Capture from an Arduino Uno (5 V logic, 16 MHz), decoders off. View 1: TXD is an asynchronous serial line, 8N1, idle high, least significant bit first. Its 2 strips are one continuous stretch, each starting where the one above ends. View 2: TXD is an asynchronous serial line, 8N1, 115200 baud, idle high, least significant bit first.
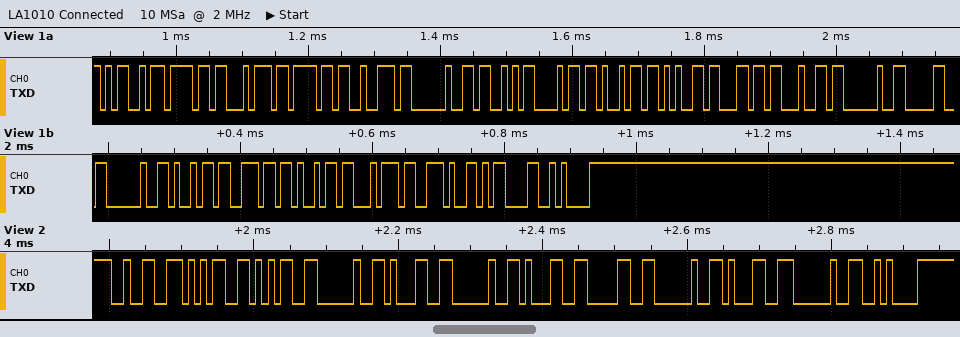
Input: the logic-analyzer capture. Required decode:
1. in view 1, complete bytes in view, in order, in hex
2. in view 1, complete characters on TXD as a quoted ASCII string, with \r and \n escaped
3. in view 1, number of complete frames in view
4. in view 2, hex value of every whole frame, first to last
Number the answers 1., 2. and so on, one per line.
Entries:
1. 4D 6F 74 6F 72 20 53 68 69 65 6C 64 20 30 20 69 6E 69 74 2E 0D 0A
2. "Motor Shield 0 init.\r\n"
3. 22
4. 32 35 35 20 31 20 31 30 20 31 20 0A
